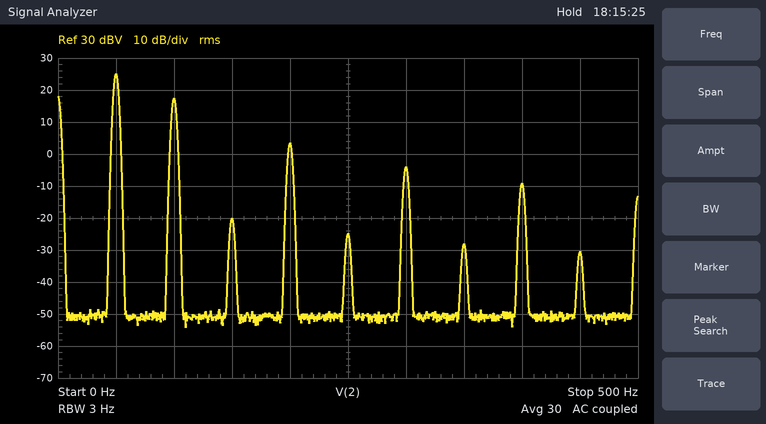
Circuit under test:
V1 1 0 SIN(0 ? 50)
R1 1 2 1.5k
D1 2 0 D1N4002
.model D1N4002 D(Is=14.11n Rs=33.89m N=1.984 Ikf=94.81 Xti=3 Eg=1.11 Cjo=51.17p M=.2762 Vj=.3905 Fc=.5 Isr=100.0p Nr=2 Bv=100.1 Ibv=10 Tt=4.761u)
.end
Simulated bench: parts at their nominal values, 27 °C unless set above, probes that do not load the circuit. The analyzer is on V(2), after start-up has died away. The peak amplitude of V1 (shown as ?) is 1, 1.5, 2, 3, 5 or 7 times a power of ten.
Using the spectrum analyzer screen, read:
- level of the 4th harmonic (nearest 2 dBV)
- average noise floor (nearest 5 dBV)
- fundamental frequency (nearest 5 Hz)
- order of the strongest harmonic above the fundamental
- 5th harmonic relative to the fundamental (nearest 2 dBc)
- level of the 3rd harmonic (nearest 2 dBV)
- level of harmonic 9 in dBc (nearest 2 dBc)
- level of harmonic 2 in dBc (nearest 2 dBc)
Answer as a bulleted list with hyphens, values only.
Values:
- 4 dBV
- -50 dBV
- 50 Hz
- 2
- -50 dBc
- -20 dBV
- -56 dBc
- -8 dBc
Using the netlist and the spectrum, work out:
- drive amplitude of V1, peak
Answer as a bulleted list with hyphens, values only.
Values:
- 50 V
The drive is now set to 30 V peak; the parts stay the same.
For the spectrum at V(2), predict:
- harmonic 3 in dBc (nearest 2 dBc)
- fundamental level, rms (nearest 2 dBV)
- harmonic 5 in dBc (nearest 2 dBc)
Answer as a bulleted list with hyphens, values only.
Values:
- -42 dBc
- 20 dBV
- -46 dBc
